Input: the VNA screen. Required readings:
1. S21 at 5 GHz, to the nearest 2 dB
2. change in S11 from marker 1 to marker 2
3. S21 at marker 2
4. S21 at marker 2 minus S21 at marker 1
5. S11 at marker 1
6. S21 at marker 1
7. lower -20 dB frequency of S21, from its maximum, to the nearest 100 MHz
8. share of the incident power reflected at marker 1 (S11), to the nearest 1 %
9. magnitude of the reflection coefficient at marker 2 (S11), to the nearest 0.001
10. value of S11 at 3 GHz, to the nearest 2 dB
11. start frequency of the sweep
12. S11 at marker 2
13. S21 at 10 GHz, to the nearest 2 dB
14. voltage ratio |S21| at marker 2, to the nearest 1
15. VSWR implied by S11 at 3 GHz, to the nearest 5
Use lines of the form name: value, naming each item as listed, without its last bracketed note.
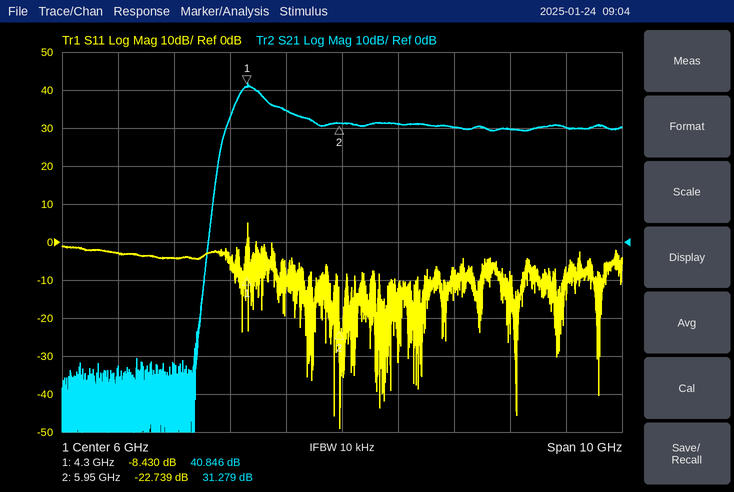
S21 at 5 GHz, to the nearest 2 dB: 34 dB
change in S11 from marker 1 to marker 2: -14.309 dB
S21 at marker 2: 31.279 dB
S21 at marker 2 minus S21 at marker 1: -9.567 dB
S11 at marker 1: -8.430 dB
S21 at marker 1: 40.846 dB
lower -20 dB frequency of S21, from its maximum, to the nearest 100 MHz: 3.8 GHz
share of the incident power reflected at marker 1 (S11), to the nearest 1 %: 14 %
magnitude of the reflection coefficient at marker 2 (S11), to the nearest 0.001: 0.073
value of S11 at 3 GHz, to the nearest 2 dB: -4 dB
start frequency of the sweep: 1 GHz
S11 at marker 2: -22.739 dB
S21 at 10 GHz, to the nearest 2 dB: 30 dB
voltage ratio |S21| at marker 2, to the nearest 1: 37
VSWR implied by S11 at 3 GHz, to the nearest 5: 5
